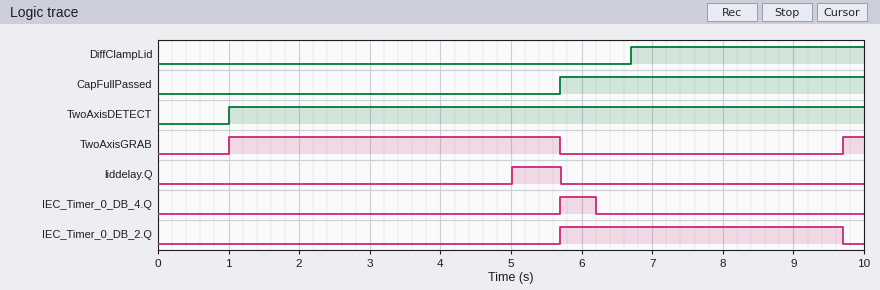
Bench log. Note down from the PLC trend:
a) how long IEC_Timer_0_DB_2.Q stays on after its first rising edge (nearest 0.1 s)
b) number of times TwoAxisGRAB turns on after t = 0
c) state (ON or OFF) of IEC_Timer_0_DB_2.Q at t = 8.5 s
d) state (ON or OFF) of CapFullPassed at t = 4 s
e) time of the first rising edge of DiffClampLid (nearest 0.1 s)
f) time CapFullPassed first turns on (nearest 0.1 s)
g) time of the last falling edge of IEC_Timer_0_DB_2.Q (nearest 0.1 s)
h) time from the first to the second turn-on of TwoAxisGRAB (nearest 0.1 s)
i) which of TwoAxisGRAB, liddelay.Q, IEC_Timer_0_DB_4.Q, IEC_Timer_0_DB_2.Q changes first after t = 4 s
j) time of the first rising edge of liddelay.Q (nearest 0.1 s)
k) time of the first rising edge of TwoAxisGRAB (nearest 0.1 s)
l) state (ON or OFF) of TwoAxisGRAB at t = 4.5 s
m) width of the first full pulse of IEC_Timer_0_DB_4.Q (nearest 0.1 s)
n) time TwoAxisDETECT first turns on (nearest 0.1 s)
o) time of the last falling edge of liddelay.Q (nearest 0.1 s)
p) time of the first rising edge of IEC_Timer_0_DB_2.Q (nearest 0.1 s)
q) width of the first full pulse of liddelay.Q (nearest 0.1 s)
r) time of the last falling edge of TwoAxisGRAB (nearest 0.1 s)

4.0 s
2
ON
OFF
6.7 s
5.7 s
9.7 s
8.7 s
liddelay.Q
5.0 s
1.0 s
ON
0.5 s
1.0 s
5.7 s
5.7 s
0.7 s
5.7 s
